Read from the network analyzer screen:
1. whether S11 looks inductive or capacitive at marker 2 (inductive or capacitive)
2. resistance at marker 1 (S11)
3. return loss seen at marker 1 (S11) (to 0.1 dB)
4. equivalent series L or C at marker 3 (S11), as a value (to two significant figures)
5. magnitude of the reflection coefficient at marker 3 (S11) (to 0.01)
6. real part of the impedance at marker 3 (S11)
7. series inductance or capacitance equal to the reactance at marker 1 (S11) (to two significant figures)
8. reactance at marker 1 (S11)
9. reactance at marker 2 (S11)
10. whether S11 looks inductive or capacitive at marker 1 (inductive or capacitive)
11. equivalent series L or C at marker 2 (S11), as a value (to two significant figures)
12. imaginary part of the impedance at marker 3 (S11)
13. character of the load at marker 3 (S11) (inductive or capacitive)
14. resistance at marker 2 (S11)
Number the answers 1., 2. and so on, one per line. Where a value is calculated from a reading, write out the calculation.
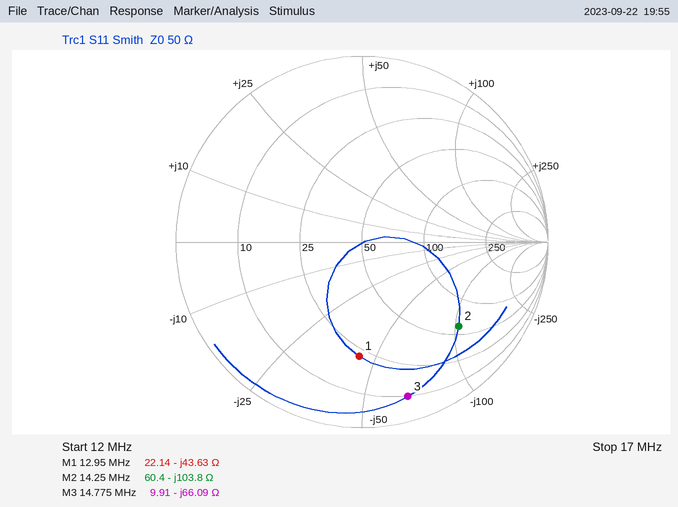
1. capacitive
2. 22.14 Ω
3. 4.2 dB
4. C = 1/(2π × 14.775 MHz × 66.09 Ω) ≈ 163 pF, so 160 pF to two significant figures
5. 0.87
6. 9.91 Ω
7. C = 1/(2π × 12.95 MHz × 43.63 Ω) ≈ 282 pF, so 280 pF to two significant figures
8. -43.63 Ω
9. -103.8 Ω
10. capacitive
11. C = 1/(2π × 14.25 MHz × 103.8 Ω) ≈ 108 pF, so 110 pF to two significant figures
12. -66.09 Ω
13. capacitive
14. 60.4 Ω
